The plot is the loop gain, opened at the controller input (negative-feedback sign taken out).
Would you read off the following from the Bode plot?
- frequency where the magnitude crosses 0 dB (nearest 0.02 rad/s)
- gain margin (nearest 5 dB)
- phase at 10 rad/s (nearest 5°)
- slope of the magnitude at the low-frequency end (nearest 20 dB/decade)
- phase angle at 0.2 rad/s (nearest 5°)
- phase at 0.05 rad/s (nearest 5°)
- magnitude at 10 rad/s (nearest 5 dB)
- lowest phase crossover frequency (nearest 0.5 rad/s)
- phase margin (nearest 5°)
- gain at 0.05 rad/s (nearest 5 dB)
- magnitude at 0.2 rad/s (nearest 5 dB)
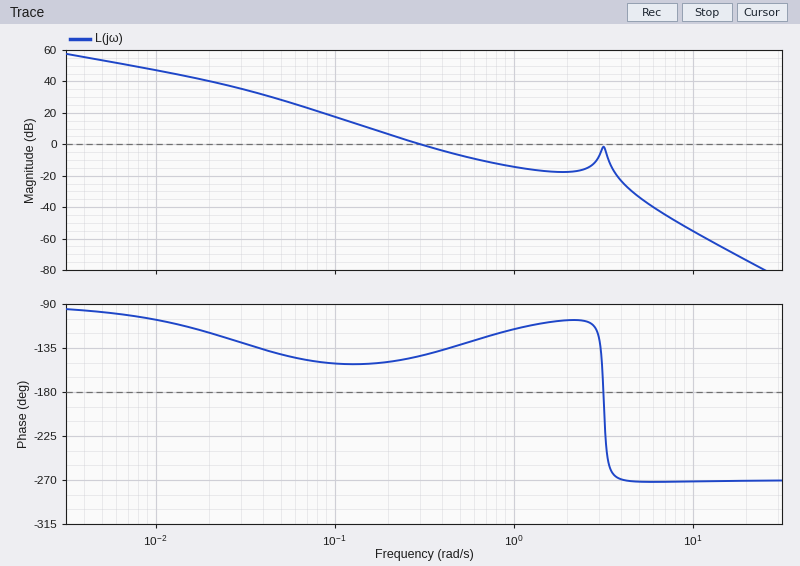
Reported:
0.30 rad/s
0 dB
-270°
-20 dB/decade
-150°
-140°
-55 dB
3.0 rad/s
35°
30 dB
5 dB
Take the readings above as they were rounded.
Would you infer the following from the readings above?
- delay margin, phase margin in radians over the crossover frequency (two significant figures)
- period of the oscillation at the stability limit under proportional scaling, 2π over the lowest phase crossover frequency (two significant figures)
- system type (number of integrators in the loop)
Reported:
2.0 s
2.1 s
1
